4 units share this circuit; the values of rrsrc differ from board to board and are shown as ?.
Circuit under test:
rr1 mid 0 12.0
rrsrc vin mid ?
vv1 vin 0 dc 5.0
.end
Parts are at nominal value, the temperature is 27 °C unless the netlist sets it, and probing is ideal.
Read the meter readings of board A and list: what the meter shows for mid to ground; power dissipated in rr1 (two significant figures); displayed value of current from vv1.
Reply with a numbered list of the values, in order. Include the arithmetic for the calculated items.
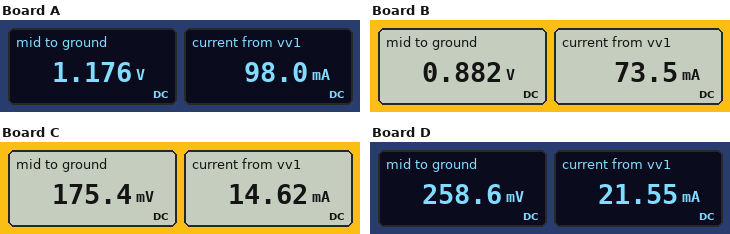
1. 1.176 V
2. (1.176 V)^2 / 12 Ω = 120 mW
3. 98.0 mA
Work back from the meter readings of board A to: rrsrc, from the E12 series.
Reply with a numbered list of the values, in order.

1. 39 Ω
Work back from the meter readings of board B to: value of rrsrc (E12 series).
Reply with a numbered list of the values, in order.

1. 56 Ω
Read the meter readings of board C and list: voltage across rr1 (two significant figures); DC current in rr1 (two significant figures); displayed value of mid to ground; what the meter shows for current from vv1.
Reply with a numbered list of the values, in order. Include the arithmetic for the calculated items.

1. 175.4 mV = 180 mV
2. (175.4 mV) / 12 Ω = 15 mA
3. 175.4 mV
4. 14.62 mA
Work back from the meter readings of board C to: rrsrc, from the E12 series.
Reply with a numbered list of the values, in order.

1. 330 Ω
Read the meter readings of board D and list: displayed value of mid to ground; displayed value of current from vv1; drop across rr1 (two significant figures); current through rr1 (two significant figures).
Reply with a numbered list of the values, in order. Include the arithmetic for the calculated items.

1. 258.6 mV
2. 21.55 mA
3. 258.6 mV = 260 mV
4. (258.6 mV) / 12 Ω = 22 mA
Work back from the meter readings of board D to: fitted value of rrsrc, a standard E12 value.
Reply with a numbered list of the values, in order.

1. 220 Ω
